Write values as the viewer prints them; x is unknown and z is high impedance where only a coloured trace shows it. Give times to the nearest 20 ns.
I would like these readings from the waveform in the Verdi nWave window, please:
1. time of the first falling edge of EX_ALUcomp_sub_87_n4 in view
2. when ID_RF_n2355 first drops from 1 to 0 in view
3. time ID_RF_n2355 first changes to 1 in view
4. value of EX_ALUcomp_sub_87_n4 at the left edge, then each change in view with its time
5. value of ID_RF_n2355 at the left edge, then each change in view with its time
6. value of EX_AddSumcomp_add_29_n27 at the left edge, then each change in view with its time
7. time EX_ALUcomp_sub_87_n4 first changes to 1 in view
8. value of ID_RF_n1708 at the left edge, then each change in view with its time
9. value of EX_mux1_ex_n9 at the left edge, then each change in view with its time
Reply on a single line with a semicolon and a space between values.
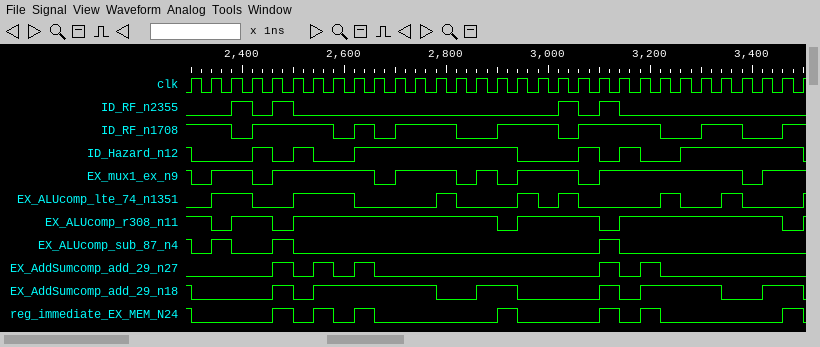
2300 ns; 2420 ns; 2380 ns; 1, 0 at 2300 ns, 1 at 2340 ns, 0 at 2380 ns, 1 at 2460 ns, 0 at 2500 ns, 1 at 3100 ns, 0 at 3140 ns; 0, 1 at 2380 ns, 0 at 2420 ns, 1 at 2460 ns, 0 at 2500 ns, 1 at 3020 ns, 0 at 3060 ns, 1 at 3100 ns, 0 at 3140 ns; 0, 1 at 2460 ns, 0 at 2500 ns, 1 at 2540 ns, 0 at 2580 ns, 1 at 2620 ns, 0 at 2660 ns, 1 at 3100 ns, 0 at 3140 ns, 1 at 3180 ns, 0 at 3220 ns; 2340 ns; 1, 0 at 2380 ns, 1 at 2420 ns, 0 at 2580 ns, 1 at 2620 ns, 0 at 2660 ns, 1 at 2700 ns, 0 at 2820 ns, 1 at 2900 ns, 0 at 3020 ns, 1 at 3060 ns, 0 at 3220 ns, 1 at 3300 ns, 0 at 3380 ns, 1 at 3460 ns; 1, 0 at 2300 ns, 1 at 2340 ns, 0 at 2420 ns, 1 at 2460 ns, 0 at 2660 ns, 1 at 2700 ns, 0 at 2820 ns, 1 at 2860 ns, 0 at 2900 ns, 1 at 2940 ns, 0 at 3060 ns, 1 at 3100 ns, 0 at 3380 ns, 1 at 3420 ns
